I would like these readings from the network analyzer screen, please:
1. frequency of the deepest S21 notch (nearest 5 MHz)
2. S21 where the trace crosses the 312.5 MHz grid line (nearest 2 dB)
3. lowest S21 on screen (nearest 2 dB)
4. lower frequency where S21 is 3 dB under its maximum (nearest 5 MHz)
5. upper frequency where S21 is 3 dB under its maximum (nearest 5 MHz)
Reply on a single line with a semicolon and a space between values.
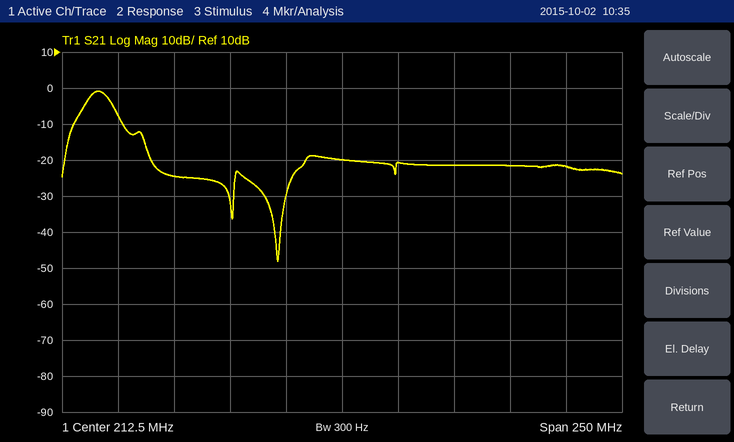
185 MHz; -22 dB; -48 dB; 100 MHz; 110 MHz
